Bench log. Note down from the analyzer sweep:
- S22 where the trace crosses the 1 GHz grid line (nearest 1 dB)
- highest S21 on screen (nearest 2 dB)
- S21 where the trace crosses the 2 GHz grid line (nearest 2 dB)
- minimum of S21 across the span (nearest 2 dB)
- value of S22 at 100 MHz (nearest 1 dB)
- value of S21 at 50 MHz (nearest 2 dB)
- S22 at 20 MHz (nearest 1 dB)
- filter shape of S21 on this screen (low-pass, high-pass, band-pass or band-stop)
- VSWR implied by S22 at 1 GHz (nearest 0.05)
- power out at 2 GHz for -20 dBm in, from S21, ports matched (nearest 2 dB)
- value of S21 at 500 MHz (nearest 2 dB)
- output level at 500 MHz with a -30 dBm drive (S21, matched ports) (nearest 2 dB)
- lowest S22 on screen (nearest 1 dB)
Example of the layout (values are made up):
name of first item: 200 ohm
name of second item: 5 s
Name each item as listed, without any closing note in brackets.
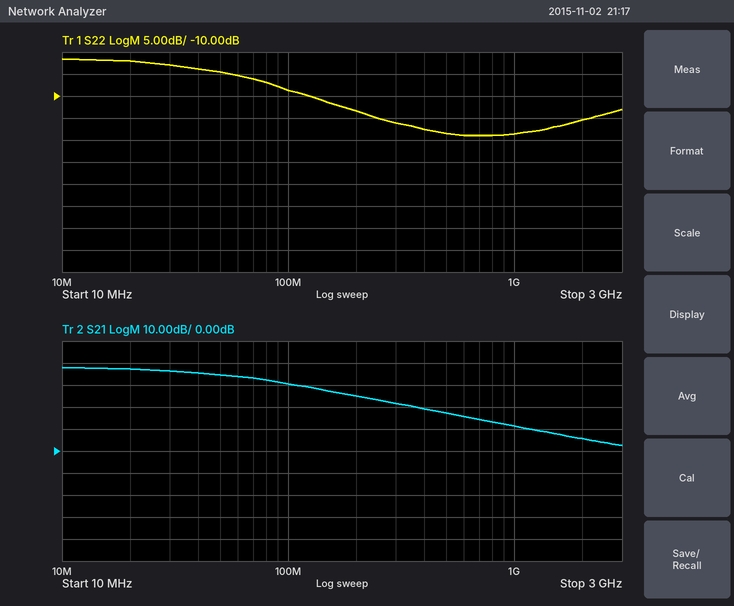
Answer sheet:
S22 where the trace crosses the 1 GHz grid line: -19 dB
highest S21 on screen: 38 dB
S21 where the trace crosses the 2 GHz grid line: 6 dB
minimum of S21 across the span: 2 dB
value of S22 at 100 MHz: -9 dB
value of S21 at 50 MHz: 34 dB
S22 at 20 MHz: -2 dB
filter shape of S21 on this screen: low-pass
VSWR implied by S22 at 1 GHz: 1.25
power out at 2 GHz for -20 dBm in, from S21, ports matched: -14 dBm
value of S21 at 500 MHz: 18 dB
output level at 500 MHz with a -30 dBm drive (S21, matched ports): -12 dBm
lowest S22 on screen: -19 dB
